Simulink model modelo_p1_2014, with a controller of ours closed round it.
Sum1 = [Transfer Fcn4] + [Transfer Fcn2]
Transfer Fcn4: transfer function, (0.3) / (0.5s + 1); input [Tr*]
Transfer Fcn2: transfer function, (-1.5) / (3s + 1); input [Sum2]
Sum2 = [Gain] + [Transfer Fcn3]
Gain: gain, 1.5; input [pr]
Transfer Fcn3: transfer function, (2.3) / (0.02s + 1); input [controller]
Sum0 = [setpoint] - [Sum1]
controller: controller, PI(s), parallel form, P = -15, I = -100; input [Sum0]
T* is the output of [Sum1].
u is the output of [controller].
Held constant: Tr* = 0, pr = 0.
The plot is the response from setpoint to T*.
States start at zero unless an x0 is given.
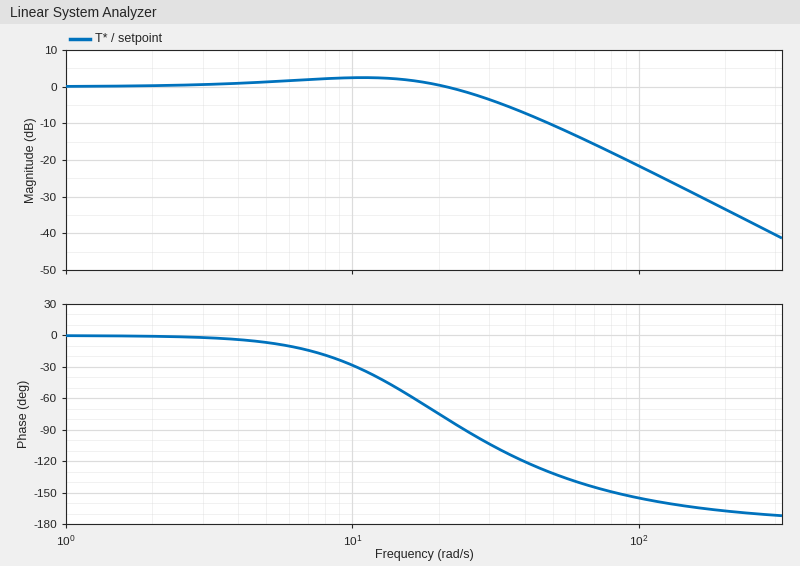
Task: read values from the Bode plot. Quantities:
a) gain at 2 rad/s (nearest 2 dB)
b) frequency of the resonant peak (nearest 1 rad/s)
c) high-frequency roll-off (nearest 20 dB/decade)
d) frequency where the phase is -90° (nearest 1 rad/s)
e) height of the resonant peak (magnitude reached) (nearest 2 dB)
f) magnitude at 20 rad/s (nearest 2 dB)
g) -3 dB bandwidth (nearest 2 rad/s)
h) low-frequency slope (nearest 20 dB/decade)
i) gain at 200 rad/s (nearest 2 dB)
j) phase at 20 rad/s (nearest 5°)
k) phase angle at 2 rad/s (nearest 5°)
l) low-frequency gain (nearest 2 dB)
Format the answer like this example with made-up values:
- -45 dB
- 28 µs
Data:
- 0 dB
- 11 rad/s
- -40 dB/decade
- 25 rad/s
- 2 dB
- 0 dB
- 28 rad/s
- 0 dB/decade
- -34 dB
- -75°
- 0°
- 0 dB
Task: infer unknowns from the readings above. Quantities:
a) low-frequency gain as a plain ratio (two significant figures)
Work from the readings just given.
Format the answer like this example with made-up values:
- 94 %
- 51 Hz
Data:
- 1.0
